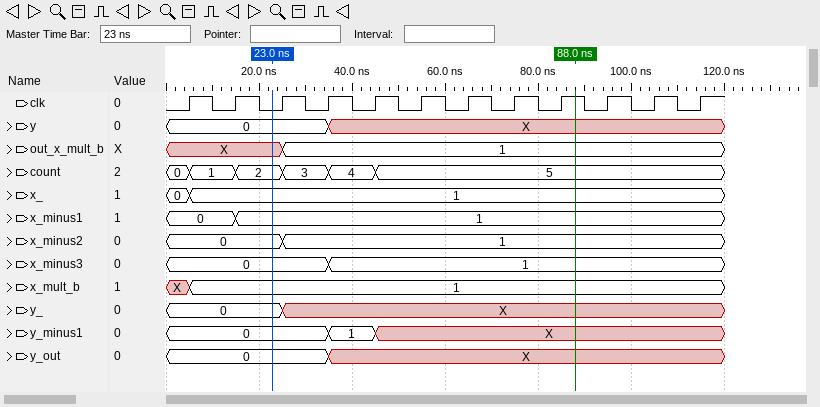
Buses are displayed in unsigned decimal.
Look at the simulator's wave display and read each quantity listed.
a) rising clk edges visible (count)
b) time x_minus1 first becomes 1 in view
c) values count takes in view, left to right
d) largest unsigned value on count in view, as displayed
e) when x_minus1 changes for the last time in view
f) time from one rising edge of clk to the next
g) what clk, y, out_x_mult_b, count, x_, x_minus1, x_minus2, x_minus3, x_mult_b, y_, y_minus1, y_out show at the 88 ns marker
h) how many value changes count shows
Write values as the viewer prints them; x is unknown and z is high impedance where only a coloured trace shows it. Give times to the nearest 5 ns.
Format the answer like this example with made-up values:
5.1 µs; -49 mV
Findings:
12; 15 ns; 0, 1, 2, 3, 4, 5; 5; 15 ns; 10 ns; clk=1, y=X, out_x_mult_b=1, count=5, x_=1, x_minus1=1, x_minus2=1, x_minus3=1, x_mult_b=1, y_=X, y_minus1=X, y_out=X; 5
